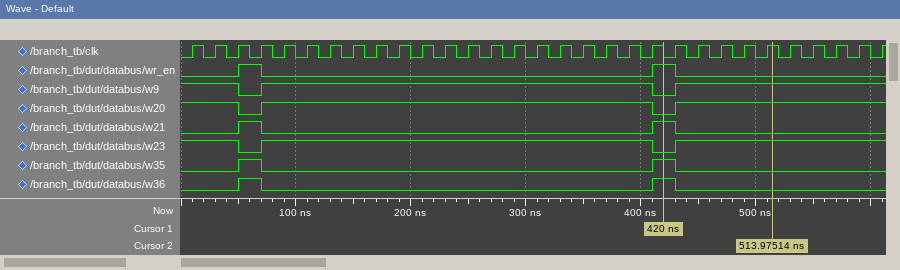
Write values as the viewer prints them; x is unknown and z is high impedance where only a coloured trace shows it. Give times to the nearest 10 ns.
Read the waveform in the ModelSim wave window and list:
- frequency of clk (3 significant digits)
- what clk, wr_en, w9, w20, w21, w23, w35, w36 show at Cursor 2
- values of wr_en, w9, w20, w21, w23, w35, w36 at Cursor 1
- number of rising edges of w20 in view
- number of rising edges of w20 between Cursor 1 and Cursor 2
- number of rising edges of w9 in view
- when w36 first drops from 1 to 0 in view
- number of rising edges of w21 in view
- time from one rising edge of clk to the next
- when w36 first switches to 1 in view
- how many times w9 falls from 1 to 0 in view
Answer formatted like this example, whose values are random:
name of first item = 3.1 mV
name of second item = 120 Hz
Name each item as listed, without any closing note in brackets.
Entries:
frequency of clk = 50.0 MHz
what clk, wr_en, w9, w20, w21, w23, w35, w36 show at Cursor 2 = clk=1, wr_en=0, w9=1, w20=1, w21=0, w23=1, w35=0, w36=0
values of wr_en, w9, w20, w21, w23, w35, w36 at Cursor 1 = wr_en=1, w9=0, w20=0, w21=1, w23=0, w35=1, w36=1
number of rising edges of w20 in view = 2
number of rising edges of w20 between Cursor 1 and Cursor 2 = 1
number of rising edges of w9 in view = 2
when w36 first drops from 1 to 0 in view = 70 ns
number of rising edges of w21 in view = 2
time from one rising edge of clk to the next = 20 ns
when w36 first switches to 1 in view = 50 ns
how many times w9 falls from 1 to 0 in view = 2
